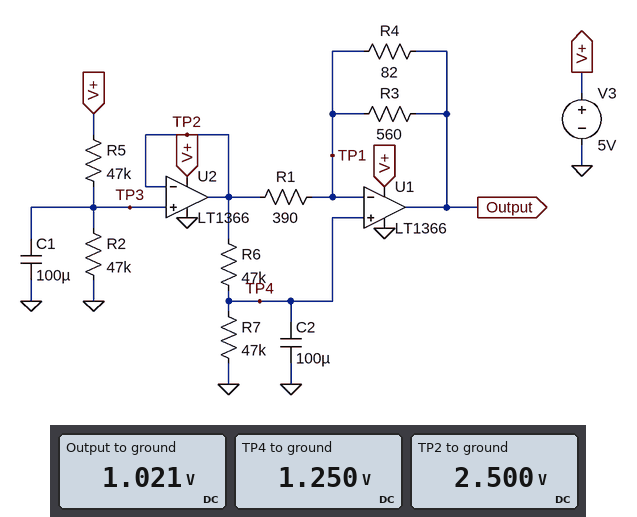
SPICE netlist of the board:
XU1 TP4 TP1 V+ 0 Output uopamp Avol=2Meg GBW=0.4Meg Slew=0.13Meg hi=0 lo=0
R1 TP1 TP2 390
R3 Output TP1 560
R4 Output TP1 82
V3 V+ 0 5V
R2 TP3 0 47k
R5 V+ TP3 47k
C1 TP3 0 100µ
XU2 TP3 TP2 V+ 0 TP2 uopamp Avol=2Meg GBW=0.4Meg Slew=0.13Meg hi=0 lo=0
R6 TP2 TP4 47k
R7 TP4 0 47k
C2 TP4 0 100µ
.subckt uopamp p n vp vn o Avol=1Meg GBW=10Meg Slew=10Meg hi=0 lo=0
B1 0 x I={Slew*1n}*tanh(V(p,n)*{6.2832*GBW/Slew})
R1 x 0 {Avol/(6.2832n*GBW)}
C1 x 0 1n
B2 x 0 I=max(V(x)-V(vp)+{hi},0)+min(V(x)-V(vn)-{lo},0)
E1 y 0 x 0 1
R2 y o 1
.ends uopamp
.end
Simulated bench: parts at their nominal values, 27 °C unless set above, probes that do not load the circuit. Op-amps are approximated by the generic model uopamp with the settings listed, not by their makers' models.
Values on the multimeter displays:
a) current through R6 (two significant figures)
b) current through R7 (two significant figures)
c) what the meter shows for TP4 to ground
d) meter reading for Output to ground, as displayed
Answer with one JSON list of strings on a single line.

["27 µA", "27 µA", "1.250 V", "1.021 V"]
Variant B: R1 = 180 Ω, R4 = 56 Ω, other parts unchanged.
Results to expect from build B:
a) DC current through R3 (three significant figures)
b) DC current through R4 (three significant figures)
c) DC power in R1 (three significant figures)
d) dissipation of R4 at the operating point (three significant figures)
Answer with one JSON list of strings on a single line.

["631 µA", "6.31 mA", "8.68 mW", "2.23 mW"]
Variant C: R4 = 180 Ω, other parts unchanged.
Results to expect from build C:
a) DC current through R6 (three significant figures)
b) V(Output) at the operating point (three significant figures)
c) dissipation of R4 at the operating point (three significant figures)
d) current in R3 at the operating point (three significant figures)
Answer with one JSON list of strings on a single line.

["26.6 µA", "813 mV", "1.06 mW", "780 µA"]
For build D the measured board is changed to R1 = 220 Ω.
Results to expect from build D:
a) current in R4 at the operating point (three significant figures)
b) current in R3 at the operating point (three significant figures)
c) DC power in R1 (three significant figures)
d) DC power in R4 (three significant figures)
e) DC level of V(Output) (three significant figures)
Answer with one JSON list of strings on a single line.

["4.96 mA", "726 µA", "7.10 mW", "2.01 mW", "844 mV"]
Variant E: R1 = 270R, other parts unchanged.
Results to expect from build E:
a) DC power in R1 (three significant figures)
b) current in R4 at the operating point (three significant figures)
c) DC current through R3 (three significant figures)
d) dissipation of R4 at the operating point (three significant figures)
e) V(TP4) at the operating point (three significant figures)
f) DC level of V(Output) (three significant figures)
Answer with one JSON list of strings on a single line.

["5.79 mW", "4.04 mA", "591 µA", "1.34 mW", "1.25 V", "919 mV"]
